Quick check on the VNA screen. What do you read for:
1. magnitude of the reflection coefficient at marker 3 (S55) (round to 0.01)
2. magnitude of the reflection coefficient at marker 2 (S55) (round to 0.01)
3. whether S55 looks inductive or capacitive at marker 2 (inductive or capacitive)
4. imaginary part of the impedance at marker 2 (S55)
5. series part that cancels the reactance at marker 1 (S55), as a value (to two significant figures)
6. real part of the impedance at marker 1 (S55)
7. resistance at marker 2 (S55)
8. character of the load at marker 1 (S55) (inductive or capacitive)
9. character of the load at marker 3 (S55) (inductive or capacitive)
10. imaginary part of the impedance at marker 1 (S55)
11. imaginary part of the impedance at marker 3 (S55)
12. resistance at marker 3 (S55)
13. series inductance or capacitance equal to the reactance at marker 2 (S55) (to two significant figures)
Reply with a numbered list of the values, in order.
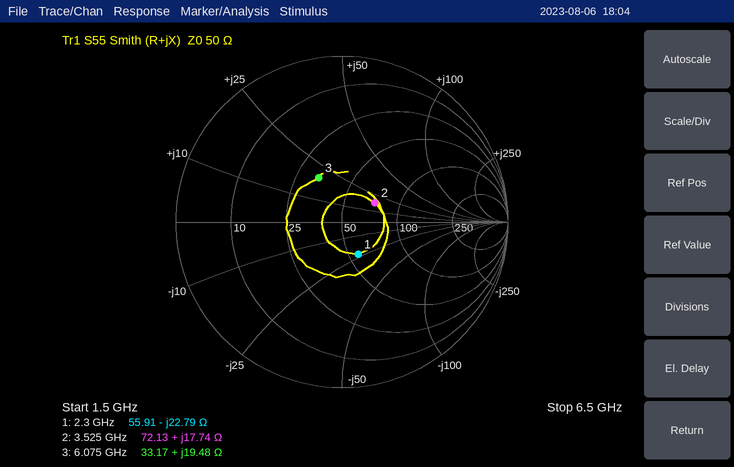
1. 0.30
2. 0.23
3. inductive
4. +17.74 Ω
5. 1.6 nH
6. 55.91 Ω
7. 72.13 Ω
8. capacitive
9. inductive
10. -22.79 Ω
11. +19.48 Ω
12. 33.17 Ω
13. 800 pH
